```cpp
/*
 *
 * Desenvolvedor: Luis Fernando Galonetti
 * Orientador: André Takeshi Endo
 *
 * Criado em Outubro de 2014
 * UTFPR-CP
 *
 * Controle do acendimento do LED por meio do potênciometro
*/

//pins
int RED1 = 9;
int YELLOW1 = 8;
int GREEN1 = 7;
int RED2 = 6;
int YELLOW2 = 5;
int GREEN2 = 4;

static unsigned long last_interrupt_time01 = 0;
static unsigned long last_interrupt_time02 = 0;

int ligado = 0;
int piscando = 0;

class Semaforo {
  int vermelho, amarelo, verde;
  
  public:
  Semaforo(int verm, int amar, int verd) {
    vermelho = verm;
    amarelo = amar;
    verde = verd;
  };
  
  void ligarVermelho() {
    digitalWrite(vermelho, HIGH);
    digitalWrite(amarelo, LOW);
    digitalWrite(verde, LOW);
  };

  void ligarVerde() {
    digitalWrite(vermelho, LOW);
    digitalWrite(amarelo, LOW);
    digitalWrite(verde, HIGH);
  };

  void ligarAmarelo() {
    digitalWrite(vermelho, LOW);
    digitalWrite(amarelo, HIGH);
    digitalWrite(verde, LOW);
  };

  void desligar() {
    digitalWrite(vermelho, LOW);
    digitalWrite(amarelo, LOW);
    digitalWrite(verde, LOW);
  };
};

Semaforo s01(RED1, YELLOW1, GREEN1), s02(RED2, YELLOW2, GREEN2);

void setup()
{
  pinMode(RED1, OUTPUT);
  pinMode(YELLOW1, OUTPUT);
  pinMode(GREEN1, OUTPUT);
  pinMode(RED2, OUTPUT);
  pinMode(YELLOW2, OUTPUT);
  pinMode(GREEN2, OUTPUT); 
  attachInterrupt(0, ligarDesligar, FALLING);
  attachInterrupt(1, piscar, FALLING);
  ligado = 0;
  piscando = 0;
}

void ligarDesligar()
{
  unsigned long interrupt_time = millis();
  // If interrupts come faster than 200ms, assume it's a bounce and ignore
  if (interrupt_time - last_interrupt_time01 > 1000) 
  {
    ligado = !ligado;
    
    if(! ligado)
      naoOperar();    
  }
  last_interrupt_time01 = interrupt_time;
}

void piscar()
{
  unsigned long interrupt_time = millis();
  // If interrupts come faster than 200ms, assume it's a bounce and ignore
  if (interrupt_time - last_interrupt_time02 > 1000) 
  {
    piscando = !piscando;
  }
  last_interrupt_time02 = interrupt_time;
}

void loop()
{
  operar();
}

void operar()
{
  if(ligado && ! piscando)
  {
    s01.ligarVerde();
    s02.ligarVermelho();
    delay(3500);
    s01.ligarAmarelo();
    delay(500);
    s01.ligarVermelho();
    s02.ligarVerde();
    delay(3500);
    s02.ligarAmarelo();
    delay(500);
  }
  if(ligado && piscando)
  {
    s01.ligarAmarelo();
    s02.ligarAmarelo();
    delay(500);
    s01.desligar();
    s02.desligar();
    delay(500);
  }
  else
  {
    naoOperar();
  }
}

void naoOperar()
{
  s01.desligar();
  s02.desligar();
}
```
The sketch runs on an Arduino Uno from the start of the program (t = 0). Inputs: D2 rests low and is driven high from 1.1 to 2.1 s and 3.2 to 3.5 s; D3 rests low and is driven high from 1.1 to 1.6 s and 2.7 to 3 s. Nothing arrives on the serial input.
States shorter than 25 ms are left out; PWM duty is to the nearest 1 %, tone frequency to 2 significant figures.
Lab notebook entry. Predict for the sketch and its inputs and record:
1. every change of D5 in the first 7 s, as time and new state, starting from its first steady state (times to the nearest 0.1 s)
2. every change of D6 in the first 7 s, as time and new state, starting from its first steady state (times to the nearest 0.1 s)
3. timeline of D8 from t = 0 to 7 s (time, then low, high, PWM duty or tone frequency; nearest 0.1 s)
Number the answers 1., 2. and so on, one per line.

1. 0 s low; 2.1 s high; 2.6 s low
2. 0 s low; 3.1 s high; 3.5 s low
3. 0 s low; 2.1 s high; 2.6 s low; 6.6 s high
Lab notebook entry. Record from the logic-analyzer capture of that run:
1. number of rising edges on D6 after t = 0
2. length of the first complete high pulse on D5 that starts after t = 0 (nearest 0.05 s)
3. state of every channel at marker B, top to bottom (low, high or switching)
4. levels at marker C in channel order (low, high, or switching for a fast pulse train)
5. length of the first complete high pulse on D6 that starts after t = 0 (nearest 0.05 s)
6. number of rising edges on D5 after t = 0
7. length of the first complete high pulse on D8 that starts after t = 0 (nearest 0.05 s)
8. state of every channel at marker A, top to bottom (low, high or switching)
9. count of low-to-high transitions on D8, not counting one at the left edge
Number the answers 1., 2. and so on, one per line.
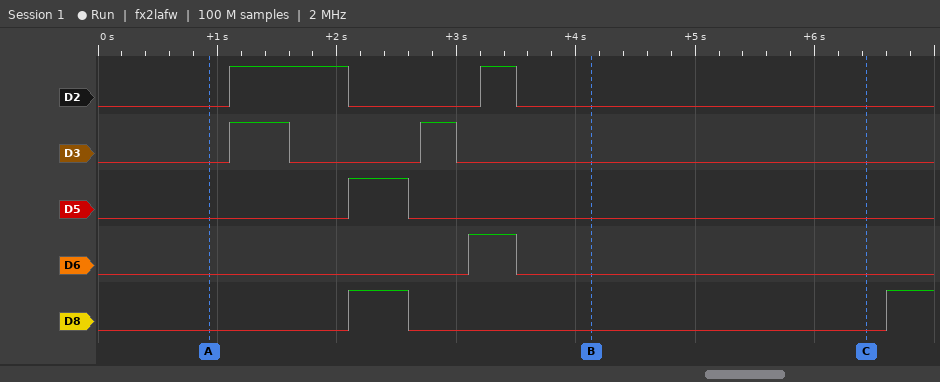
1. 1
2. 0.50 s
3. D2 low, D3 low, D5 low, D6 low, D8 low
4. D2 low, D3 low, D5 low, D6 low, D8 low
5. 0.40 s
6. 1
7. 0.50 s
8. D2 low, D3 low, D5 low, D6 low, D8 low
9. 2
